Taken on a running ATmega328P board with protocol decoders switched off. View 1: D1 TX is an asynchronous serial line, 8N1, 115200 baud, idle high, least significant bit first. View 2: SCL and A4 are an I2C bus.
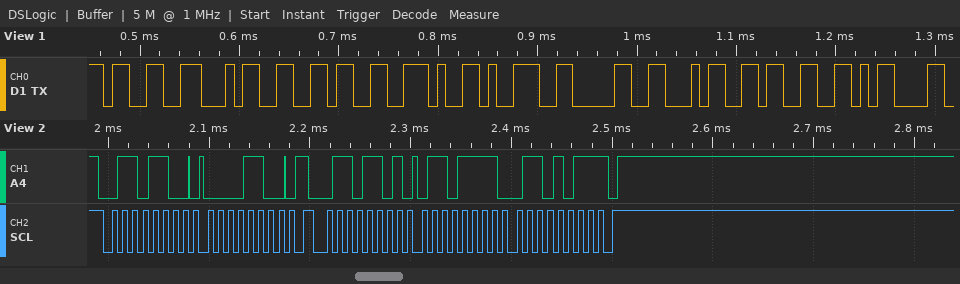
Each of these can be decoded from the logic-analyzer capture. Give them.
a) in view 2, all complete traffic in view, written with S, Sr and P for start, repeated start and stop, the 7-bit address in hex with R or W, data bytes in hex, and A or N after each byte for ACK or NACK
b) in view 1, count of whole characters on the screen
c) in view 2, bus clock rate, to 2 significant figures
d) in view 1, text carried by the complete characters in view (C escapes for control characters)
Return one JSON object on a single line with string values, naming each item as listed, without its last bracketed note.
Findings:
{"in view 2, all complete traffic in view, written with S, Sr and P for start, repeated start and stop, the 7-bit address in hex with R or W, data bytes in hex, and A or N after each byte for ACK or NACK": "S 36W A 0C A Sr 36R A 6F A 6B N P", "in view 1, count of whole characters on the screen": "9", "in view 2, bus clock rate, to 2 significant figures": "100 kHz", "in view 1, text carried by the complete characters in view": "\"346.9043\\r\""}
